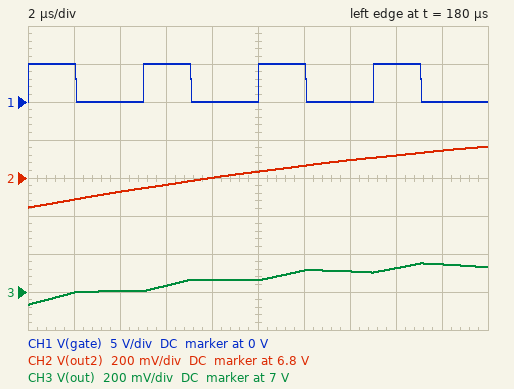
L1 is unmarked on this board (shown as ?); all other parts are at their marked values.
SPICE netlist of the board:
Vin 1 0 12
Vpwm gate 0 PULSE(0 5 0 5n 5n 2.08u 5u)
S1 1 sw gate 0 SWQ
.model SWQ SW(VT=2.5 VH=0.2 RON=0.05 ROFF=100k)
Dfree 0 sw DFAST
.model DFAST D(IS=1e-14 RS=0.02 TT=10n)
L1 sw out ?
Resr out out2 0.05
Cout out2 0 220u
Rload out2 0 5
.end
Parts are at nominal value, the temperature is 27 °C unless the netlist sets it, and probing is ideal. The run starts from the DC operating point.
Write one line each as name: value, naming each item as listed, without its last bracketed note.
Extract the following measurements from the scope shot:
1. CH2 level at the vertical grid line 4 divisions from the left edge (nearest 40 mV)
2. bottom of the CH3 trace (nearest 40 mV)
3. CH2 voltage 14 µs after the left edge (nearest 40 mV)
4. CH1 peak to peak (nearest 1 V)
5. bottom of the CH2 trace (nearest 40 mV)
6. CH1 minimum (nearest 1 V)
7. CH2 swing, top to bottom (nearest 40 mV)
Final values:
CH2 level at the vertical grid line 4 divisions from the left edge: 6.80 V
bottom of the CH3 trace: 6.92 V
CH2 voltage 14 µs after the left edge: 6.88 V
CH1 peak to peak: 5 V
bottom of the CH2 trace: 6.64 V
CH1 minimum: 0 V
CH2 swing, top to bottom: 320 mV
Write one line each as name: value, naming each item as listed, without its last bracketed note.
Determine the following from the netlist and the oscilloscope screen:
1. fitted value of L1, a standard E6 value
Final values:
fitted value of L1, a standard E6 value: 22 µH
